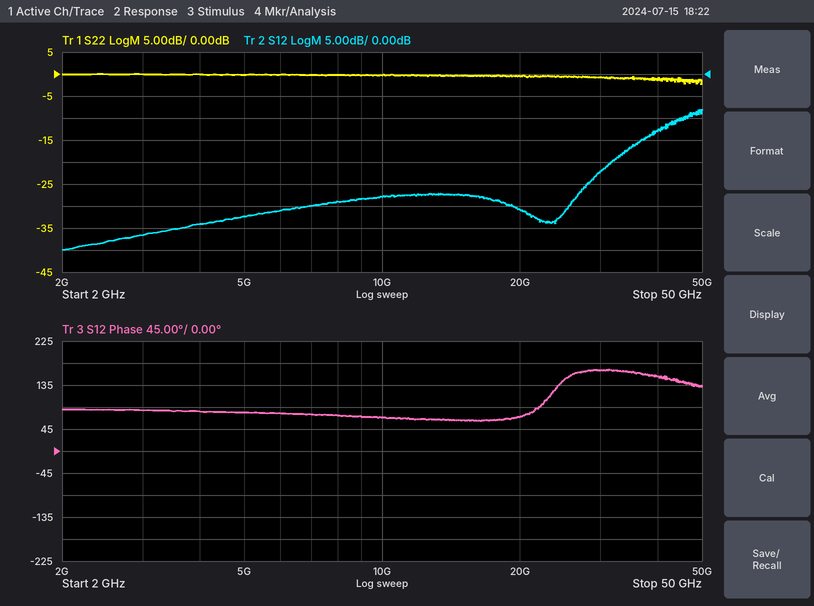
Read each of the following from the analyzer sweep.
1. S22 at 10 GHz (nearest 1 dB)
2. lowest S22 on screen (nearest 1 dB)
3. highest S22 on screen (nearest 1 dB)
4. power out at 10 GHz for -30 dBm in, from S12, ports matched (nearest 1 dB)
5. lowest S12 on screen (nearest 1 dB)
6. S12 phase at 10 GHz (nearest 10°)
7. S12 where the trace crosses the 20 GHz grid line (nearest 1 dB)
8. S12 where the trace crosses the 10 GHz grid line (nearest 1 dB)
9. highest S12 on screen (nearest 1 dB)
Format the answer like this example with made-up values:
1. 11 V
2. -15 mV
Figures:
1. 0 dB
2. -2 dB
3. 0 dB
4. -58 dBm
5. -40 dB
6. 70°
7. -31 dB
8. -28 dB
9. -8 dB
